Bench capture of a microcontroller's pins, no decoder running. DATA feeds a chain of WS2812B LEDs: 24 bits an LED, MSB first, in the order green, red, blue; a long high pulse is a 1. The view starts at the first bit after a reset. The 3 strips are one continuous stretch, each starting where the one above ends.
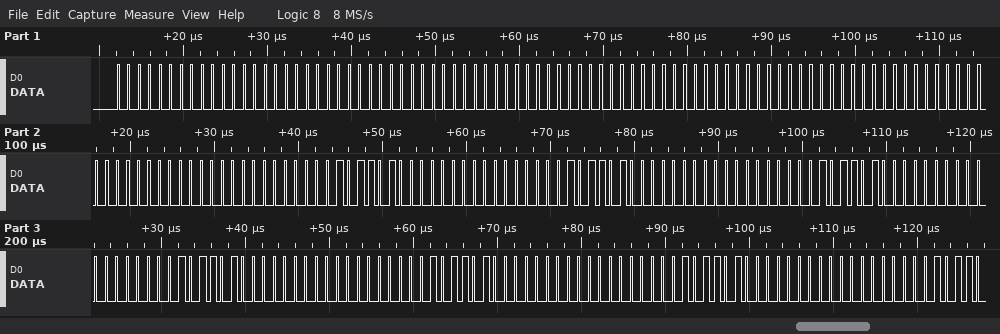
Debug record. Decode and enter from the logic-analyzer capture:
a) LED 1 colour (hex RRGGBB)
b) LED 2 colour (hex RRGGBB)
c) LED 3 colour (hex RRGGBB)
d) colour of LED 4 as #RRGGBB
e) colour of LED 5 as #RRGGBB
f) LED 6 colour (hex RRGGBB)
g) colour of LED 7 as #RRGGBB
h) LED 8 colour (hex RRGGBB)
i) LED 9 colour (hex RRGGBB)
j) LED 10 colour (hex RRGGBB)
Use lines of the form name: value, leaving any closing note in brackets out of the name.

LED 1 colour: #000000
LED 2 colour: #000000
LED 3 colour: #000000
colour of LED 4 as #RRGGBB: #000000
colour of LED 5 as #RRGGBB: #2D0000
LED 6 colour: #B40000
colour of LED 7 as #RRGGBB: #B40000
LED 8 colour: #B40000
LED 9 colour: #B40000
LED 10 colour: #B40000
